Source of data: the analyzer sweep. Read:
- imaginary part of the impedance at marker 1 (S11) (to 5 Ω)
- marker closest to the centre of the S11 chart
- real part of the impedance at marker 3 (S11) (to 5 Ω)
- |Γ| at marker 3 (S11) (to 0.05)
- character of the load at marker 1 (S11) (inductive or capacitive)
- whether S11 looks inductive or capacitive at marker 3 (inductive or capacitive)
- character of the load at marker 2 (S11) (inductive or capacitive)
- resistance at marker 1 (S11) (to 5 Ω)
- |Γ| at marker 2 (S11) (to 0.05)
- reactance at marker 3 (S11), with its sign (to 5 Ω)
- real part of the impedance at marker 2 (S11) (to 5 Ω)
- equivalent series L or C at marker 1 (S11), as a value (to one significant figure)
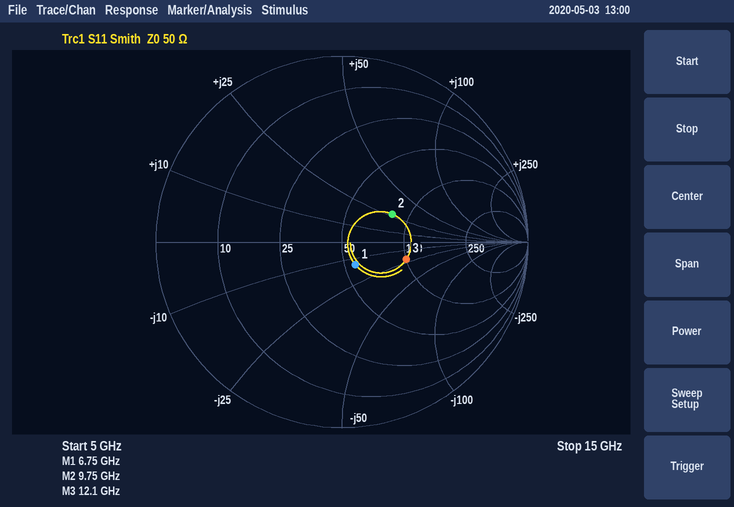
-15 Ω
marker 1
100 Ω
0.35
capacitive
capacitive
inductive
55 Ω
0.30
-20 Ω
80 Ω
2 pF
